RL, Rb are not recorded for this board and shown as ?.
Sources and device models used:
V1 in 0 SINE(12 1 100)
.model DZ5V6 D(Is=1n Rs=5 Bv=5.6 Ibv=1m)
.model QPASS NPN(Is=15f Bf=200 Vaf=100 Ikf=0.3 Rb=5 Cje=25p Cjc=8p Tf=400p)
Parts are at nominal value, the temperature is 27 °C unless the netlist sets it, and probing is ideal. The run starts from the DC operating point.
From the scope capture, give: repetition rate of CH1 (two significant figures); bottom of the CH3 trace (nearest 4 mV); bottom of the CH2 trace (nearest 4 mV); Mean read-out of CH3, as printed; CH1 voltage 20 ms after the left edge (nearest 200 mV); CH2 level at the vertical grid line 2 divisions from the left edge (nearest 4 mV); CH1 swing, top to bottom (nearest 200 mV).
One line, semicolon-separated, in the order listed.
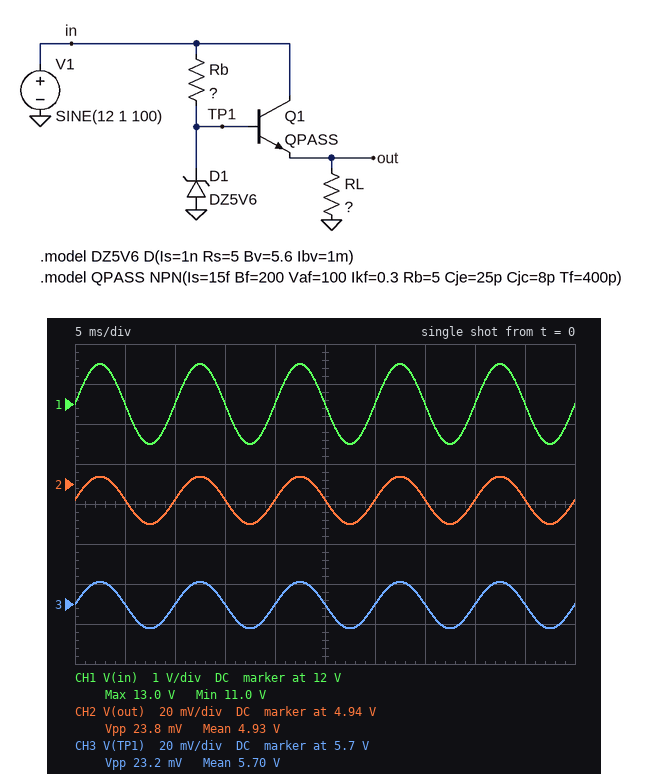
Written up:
100 Hz; 5.688 V; 4.920 V; 5.70 V; 12.0 V; 4.932 V; 2.0 V
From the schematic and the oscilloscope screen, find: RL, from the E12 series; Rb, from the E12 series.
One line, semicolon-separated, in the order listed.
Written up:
56 Ω; 680 Ω
